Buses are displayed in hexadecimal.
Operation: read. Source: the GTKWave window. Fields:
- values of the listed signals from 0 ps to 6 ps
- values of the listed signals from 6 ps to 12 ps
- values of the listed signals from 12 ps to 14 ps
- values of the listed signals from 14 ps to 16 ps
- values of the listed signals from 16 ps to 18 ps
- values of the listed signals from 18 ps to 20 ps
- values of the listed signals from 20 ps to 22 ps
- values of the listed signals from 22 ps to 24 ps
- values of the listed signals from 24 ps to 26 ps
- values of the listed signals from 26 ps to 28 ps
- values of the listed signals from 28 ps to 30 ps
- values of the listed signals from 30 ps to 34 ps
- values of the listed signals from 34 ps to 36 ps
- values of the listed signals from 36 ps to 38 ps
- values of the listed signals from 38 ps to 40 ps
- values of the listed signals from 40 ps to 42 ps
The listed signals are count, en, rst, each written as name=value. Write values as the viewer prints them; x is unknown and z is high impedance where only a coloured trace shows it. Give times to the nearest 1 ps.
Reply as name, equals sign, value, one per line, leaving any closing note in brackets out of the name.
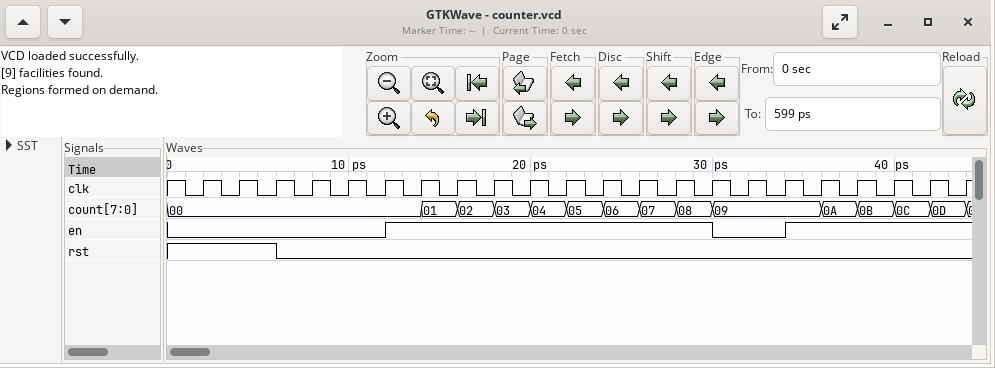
values of the listed signals from 0 ps to 6 ps = count=00, en=0, rst=1
values of the listed signals from 6 ps to 12 ps = count=00, en=0, rst=0
values of the listed signals from 12 ps to 14 ps = count=00, en=1, rst=0
values of the listed signals from 14 ps to 16 ps = count=01, en=1, rst=0
values of the listed signals from 16 ps to 18 ps = count=02, en=1, rst=0
values of the listed signals from 18 ps to 20 ps = count=03, en=1, rst=0
values of the listed signals from 20 ps to 22 ps = count=04, en=1, rst=0
values of the listed signals from 22 ps to 24 ps = count=05, en=1, rst=0
values of the listed signals from 24 ps to 26 ps = count=06, en=1, rst=0
values of the listed signals from 26 ps to 28 ps = count=07, en=1, rst=0
values of the listed signals from 28 ps to 30 ps = count=08, en=1, rst=0
values of the listed signals from 30 ps to 34 ps = count=09, en=0, rst=0
values of the listed signals from 34 ps to 36 ps = count=09, en=1, rst=0
values of the listed signals from 36 ps to 38 ps = count=0A, en=1, rst=0
values of the listed signals from 38 ps to 40 ps = count=0B, en=1, rst=0
values of the listed signals from 40 ps to 42 ps = count=0C, en=1, rst=0
